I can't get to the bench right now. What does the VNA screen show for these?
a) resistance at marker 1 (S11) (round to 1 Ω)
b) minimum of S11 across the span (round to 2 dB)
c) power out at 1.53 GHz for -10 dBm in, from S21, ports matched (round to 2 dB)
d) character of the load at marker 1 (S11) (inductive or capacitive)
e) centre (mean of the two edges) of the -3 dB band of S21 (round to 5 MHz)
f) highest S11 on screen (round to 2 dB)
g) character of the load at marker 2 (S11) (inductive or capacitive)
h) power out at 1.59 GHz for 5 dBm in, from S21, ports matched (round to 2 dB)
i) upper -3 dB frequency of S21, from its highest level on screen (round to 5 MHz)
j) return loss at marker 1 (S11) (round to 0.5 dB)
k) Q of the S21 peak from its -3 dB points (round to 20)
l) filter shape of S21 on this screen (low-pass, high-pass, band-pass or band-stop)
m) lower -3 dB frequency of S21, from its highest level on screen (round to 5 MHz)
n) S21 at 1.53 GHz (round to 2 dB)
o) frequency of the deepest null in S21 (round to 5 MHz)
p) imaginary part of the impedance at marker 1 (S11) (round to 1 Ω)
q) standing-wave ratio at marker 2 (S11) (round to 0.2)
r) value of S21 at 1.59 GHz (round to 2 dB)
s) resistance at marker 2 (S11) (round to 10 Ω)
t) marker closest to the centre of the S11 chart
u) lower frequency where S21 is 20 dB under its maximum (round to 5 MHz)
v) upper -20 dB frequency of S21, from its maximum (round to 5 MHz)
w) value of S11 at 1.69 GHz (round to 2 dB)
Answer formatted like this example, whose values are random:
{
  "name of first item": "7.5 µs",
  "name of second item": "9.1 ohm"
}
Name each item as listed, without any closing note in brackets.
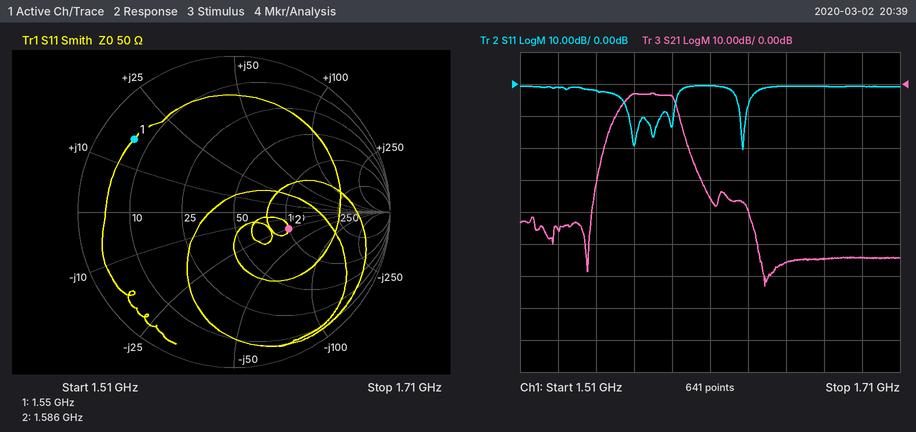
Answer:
{
  "resistance at marker 1 (S11)": "6 Ω",
  "minimum of S11 across the span": "-20 dB",
  "power out at 1.53 GHz for -10 dBm in, from S21, ports matched": "-56 dBm",
  "character of the load at marker 1 (S11)": "inductive",
  "centre (mean of the two edges) of the -3 dB band of S21": "1.580 GHz",
  "highest S11 on screen": "0 dB",
  "character of the load at marker 2 (S11)": "capacitive",
  "power out at 1.59 GHz for 5 dBm in, from S21, ports matched": "2 dBm",
  "upper -3 dB frequency of S21, from its highest level on screen": "1.590 GHz",
  "return loss at marker 1 (S11)": "2.0 dB",
  "Q of the S21 peak from its -3 dB points": "60",
  "filter shape of S21 on this screen": "band-pass",
  "lower -3 dB frequency of S21, from its highest level on screen": "1.565 GHz",
  "S21 at 1.53 GHz": "-46 dB",
  "frequency of the deepest null in S21": "1.640 GHz",
  "imaginary part of the impedance at marker 1 (S11)": "+16 Ω",
  "standing-wave ratio at marker 2 (S11)": "2.2",
  "value of S21 at 1.59 GHz": "-4 dB",
  "resistance at marker 2 (S11)": "100 Ω",
  "marker closest to the centre of the S11 chart": "marker 2",
  "lower frequency where S21 is 20 dB under its maximum": "1.555 GHz",
  "upper -20 dB frequency of S21, from its maximum": "1.600 GHz",
  "value of S11 at 1.69 GHz": "0 dB"
}
